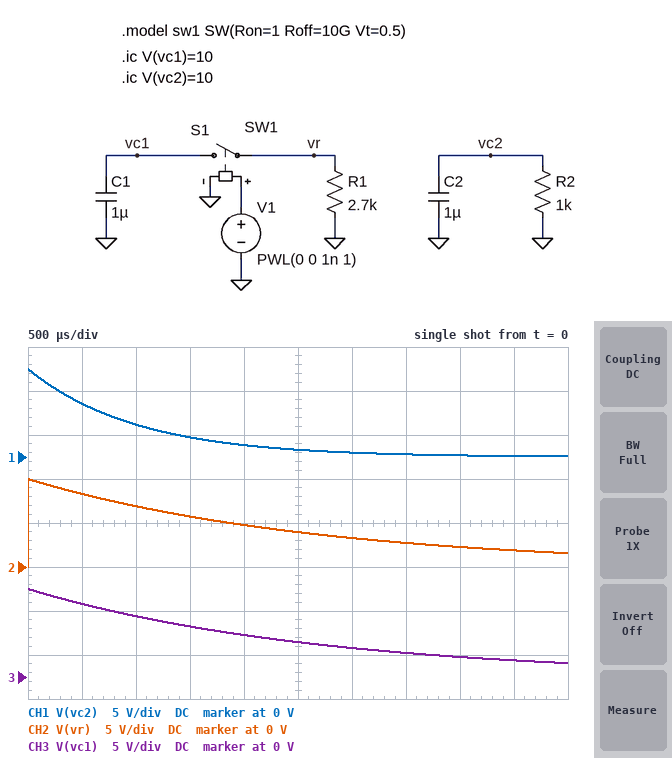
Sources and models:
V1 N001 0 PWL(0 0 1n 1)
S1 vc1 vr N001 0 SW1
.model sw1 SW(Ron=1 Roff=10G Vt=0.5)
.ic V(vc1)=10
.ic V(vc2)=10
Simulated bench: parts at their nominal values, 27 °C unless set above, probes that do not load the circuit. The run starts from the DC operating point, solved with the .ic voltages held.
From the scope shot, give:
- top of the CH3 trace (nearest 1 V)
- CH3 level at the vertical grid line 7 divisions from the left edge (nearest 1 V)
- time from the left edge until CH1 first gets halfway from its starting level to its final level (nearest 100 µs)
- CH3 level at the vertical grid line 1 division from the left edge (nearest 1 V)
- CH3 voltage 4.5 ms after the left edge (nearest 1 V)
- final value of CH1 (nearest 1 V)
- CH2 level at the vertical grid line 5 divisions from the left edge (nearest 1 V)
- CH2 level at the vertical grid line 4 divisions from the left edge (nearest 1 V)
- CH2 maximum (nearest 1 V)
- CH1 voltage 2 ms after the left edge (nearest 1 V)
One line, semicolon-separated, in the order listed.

10 V; 3 V; 700 µs; 8 V; 2 V; 0 V; 4 V; 5 V; 10 V; 1 V
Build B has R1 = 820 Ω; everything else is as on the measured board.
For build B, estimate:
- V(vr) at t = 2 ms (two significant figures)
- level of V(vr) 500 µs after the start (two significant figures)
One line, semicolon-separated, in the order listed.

870 mV; 5.4 V
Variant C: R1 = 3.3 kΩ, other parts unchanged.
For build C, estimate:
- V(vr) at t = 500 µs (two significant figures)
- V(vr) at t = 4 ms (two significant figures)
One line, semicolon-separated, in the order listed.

8.6 V; 3.0 V
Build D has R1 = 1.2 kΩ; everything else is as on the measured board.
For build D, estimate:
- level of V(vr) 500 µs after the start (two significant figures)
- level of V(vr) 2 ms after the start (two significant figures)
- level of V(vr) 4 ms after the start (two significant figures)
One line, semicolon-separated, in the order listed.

6.6 V; 1.9 V; 360 mV
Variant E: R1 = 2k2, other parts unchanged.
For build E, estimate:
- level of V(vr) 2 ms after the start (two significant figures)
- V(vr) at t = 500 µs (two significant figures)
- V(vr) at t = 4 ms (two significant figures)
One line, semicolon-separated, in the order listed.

4.0 V; 8.0 V; 1.6 V
